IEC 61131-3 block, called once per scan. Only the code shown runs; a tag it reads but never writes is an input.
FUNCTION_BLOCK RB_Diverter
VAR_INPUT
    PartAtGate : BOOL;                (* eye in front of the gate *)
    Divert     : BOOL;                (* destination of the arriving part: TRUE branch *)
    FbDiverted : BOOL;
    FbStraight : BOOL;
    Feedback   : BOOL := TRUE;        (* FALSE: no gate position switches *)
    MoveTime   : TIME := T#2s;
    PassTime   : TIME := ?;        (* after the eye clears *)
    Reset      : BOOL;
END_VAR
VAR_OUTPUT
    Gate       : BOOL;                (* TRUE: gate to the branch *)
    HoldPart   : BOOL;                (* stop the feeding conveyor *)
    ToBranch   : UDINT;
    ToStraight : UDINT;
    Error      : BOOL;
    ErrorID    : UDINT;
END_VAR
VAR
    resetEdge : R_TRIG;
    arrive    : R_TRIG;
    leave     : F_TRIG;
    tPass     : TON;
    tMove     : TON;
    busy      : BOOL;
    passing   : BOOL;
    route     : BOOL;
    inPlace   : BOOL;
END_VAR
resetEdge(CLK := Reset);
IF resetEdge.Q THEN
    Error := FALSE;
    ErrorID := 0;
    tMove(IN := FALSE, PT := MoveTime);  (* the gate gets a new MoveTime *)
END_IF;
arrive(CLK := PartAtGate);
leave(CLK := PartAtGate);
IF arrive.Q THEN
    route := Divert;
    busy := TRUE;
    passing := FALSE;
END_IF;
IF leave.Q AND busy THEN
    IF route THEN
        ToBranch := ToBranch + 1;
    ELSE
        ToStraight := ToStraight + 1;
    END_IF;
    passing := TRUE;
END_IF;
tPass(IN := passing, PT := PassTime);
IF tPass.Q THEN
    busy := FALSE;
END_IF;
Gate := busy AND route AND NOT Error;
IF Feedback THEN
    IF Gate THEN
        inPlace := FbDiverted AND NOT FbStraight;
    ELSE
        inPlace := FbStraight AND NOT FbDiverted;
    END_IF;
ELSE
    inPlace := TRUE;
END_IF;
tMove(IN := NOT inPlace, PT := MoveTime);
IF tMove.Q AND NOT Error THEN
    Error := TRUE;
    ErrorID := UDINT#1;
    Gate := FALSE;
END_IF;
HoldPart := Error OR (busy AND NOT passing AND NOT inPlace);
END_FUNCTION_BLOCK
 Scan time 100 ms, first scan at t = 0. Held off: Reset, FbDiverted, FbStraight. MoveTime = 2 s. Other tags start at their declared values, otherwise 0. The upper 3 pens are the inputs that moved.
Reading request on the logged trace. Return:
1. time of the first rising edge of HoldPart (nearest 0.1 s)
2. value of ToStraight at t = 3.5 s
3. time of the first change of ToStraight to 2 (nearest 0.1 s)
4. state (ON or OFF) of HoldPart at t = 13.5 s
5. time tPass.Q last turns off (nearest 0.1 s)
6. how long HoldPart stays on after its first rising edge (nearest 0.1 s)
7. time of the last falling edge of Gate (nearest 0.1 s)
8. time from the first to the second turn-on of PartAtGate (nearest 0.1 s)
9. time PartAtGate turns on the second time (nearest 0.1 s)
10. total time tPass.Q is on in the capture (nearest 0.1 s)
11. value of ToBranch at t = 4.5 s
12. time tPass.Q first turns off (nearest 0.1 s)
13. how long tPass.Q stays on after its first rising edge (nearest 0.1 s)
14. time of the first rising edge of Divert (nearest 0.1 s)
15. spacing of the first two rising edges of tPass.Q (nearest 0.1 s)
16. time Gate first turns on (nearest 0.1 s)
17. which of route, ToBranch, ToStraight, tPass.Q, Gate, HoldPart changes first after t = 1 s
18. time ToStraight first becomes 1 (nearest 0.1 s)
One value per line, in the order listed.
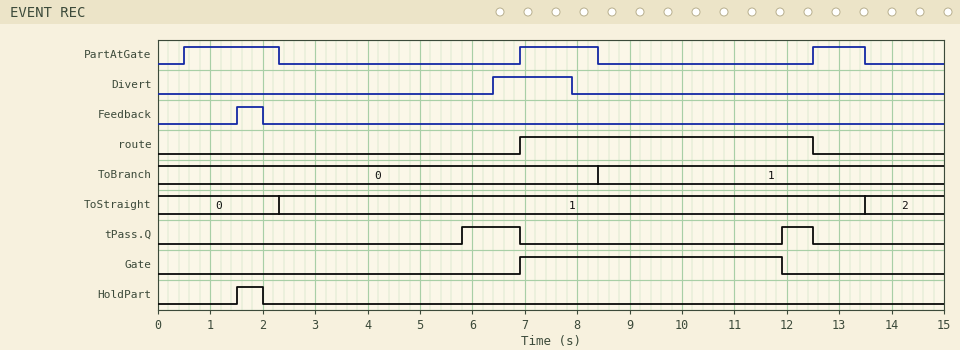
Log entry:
1.5 s
1
13.5 s
OFF
12.5 s
0.5 s
11.9 s
6.4 s
6.9 s
1.7 s
0
6.9 s
1.1 s
6.4 s
6.1 s
6.9 s
HoldPart
2.3 s
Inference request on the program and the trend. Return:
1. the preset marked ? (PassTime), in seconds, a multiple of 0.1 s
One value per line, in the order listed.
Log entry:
3.5 s
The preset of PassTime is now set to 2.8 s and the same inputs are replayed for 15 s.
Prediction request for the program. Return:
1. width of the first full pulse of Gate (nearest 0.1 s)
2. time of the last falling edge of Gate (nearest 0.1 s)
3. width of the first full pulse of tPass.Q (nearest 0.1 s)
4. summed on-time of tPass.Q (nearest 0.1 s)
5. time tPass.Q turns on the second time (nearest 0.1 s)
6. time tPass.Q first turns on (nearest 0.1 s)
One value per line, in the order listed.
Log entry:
4.3 s
11.2 s
1.8 s
3.1 s
11.2 s
5.1 s
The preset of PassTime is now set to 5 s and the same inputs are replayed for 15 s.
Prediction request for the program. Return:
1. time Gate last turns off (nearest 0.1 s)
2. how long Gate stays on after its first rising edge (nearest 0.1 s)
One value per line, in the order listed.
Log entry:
12.5 s
5.6 s
